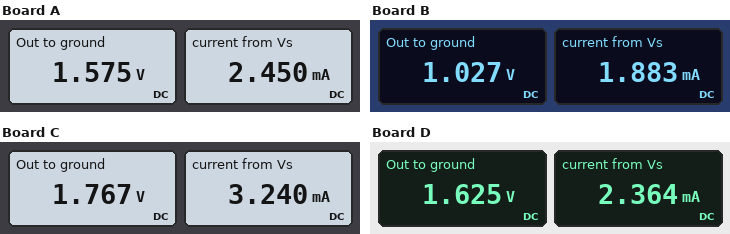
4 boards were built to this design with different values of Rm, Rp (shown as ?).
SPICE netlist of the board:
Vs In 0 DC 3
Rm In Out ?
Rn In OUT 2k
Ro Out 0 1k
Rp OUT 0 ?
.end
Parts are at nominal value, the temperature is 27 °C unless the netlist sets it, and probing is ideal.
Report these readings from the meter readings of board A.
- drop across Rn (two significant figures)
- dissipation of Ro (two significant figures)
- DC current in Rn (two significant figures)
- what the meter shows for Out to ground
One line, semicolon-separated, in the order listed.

1.4 V; 2.5 mW; 710 µA; 1.575 V
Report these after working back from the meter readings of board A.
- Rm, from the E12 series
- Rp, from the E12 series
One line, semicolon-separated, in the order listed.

820 Ω; 1.8 kΩ
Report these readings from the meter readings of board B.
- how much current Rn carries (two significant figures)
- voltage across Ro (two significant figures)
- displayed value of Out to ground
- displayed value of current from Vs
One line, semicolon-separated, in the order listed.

990 µA; 1.0 V; 1.027 V; 1.883 mA
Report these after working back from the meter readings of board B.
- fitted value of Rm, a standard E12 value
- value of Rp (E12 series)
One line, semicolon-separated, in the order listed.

2.2 kΩ; 1.2 kΩ
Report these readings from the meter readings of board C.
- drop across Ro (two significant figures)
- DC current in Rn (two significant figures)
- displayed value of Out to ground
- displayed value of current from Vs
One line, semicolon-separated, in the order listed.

1.8 V; 620 µA; 1.767 V; 3.240 mA
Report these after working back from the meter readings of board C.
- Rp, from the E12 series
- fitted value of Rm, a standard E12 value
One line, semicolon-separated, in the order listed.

1.2 kΩ; 470 Ω
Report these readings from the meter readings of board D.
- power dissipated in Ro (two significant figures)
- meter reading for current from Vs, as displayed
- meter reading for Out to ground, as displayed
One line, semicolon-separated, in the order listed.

2.6 mW; 2.364 mA; 1.625 V
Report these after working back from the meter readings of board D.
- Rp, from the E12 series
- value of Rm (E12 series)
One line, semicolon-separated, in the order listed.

2.2 kΩ; 820 Ω
